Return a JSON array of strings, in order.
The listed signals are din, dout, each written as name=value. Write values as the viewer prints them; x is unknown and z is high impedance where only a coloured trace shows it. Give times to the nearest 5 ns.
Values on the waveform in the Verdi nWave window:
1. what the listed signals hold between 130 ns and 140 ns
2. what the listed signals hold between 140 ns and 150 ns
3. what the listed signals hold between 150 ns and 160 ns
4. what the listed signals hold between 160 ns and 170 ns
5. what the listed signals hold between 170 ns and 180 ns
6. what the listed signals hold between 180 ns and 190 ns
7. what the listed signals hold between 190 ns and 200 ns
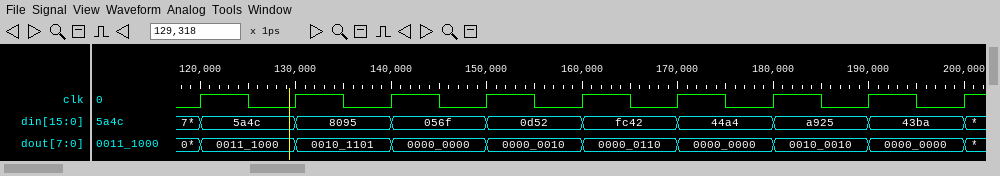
["din=8095, dout=0010_1101", "din=056f, dout=0000_0000", "din=0d52, dout=0000_0010", "din=fc42, dout=0000_0110", "din=44a4, dout=0000_0000", "din=a925, dout=0010_0010", "din=43ba, dout=0000_0000"]
